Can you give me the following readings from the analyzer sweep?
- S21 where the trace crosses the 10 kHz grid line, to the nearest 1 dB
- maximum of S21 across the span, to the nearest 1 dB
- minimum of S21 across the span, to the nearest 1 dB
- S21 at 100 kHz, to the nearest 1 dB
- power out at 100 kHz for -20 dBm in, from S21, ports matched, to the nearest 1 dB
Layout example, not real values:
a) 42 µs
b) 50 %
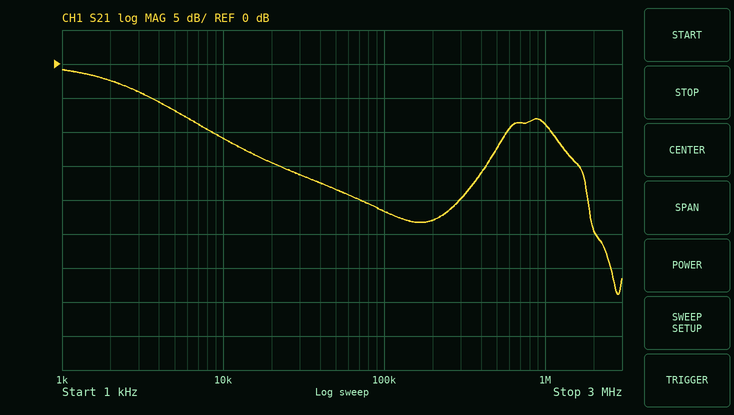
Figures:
a) -11 dB
b) -1 dB
c) -34 dB
d) -22 dB
e) -42 dBm
